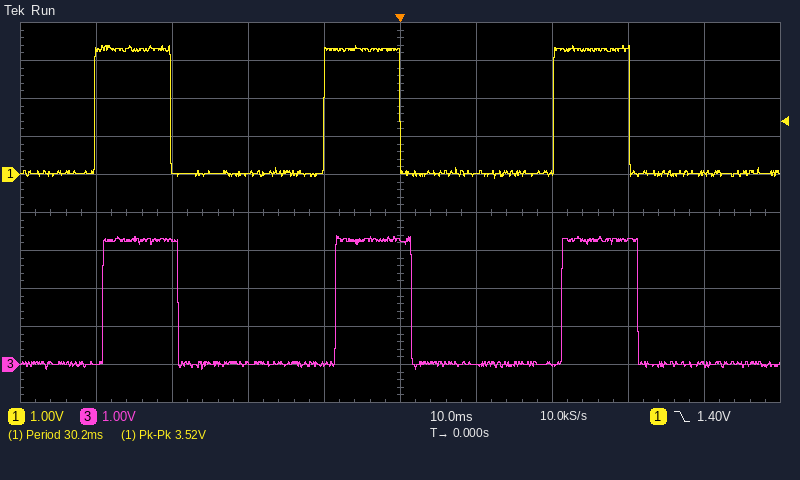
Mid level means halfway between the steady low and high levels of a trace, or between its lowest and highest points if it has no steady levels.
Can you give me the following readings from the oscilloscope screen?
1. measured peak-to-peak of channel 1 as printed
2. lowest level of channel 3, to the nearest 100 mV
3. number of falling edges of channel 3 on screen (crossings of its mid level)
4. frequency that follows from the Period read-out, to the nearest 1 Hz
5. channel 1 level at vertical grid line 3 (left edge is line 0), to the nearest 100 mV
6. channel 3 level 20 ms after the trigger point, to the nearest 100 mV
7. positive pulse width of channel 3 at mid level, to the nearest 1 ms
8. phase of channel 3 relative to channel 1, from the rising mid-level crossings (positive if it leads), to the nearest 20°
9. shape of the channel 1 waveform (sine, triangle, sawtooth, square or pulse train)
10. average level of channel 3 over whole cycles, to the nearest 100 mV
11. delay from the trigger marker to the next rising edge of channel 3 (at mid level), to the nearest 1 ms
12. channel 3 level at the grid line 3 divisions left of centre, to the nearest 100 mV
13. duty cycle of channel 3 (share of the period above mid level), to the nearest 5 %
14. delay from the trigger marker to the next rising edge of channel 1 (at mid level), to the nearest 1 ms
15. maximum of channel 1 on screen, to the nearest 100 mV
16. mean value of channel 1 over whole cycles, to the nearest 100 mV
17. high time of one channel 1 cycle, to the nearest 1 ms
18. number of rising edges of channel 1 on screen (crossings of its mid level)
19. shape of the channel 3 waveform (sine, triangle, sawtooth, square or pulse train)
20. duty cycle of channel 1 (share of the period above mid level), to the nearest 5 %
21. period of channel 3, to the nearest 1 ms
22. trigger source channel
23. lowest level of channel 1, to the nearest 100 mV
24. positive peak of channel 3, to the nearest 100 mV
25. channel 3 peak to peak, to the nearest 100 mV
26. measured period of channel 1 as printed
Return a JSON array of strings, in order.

["3.52 V", "-100 mV", "3", "33 Hz", "0.0 V", "0.0 V", "10 ms", "-20°", "pulse train", "1.1 V", "21 ms", "3.3 V", "35 %", "20 ms", "3.4 V", "1.1 V", "10 ms", "3", "pulse train", "35 %", "30 ms", "channel 1", "-100 mV", "3.4 V", "3.5 V", "30.2 ms"]
